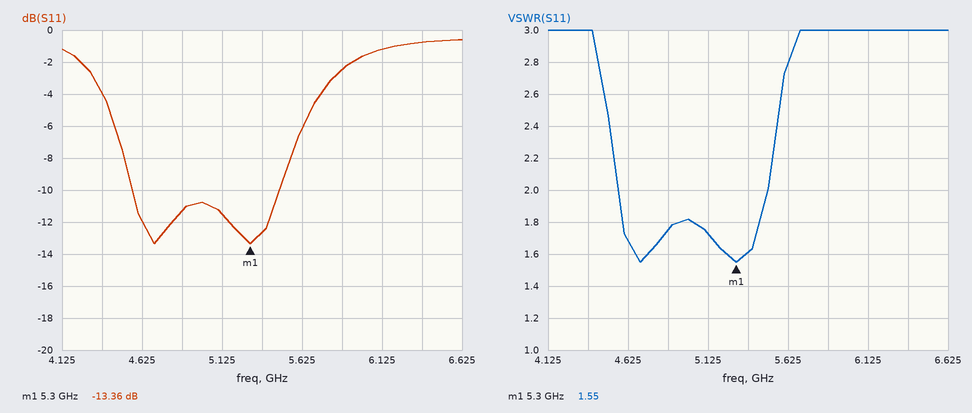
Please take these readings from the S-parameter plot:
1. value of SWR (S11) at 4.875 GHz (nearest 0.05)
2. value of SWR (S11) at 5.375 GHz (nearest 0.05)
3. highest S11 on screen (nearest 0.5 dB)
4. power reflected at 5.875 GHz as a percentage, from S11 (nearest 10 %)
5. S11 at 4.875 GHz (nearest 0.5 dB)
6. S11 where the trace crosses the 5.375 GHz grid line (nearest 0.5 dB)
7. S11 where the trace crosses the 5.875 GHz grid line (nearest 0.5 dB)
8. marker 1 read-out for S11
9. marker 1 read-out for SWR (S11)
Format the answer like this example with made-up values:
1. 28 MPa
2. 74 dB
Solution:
1. 1.75
2. 1.60
3. -0.5 dB
4. 60 %
5. -11.5 dB
6. -12.5 dB
7. -2.5 dB
8. -13.36 dB
9. 1.55
